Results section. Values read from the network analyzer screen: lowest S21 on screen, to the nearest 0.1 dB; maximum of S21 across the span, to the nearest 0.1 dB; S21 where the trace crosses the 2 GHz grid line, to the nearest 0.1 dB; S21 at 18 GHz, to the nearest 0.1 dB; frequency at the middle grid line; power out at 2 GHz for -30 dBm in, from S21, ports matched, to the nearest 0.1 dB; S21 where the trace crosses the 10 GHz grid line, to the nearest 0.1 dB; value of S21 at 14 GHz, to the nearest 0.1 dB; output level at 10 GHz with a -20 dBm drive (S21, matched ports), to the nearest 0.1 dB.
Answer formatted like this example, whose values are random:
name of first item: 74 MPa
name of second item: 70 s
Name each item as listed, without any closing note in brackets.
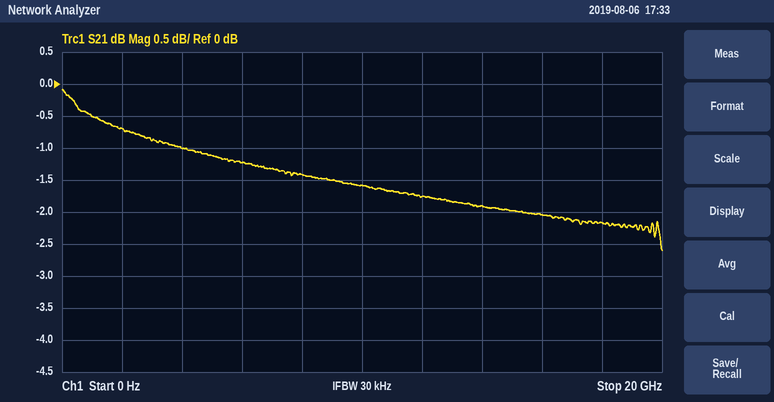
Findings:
lowest S21 on screen, to the nearest 0.1 dB: -2.6 dB
maximum of S21 across the span, to the nearest 0.1 dB: -0.1 dB
S21 where the trace crosses the 2 GHz grid line, to the nearest 0.1 dB: -0.7 dB
S21 at 18 GHz, to the nearest 0.1 dB: -2.2 dB
frequency at the middle grid line: 10 GHz
power out at 2 GHz for -30 dBm in, from S21, ports matched, to the nearest 0.1 dB: -30.7 dBm
S21 where the trace crosses the 10 GHz grid line, to the nearest 0.1 dB: -1.6 dB
value of S21 at 14 GHz, to the nearest 0.1 dB: -1.9 dB
output level at 10 GHz with a -20 dBm drive (S21, matched ports), to the nearest 0.1 dB: -21.6 dBm
